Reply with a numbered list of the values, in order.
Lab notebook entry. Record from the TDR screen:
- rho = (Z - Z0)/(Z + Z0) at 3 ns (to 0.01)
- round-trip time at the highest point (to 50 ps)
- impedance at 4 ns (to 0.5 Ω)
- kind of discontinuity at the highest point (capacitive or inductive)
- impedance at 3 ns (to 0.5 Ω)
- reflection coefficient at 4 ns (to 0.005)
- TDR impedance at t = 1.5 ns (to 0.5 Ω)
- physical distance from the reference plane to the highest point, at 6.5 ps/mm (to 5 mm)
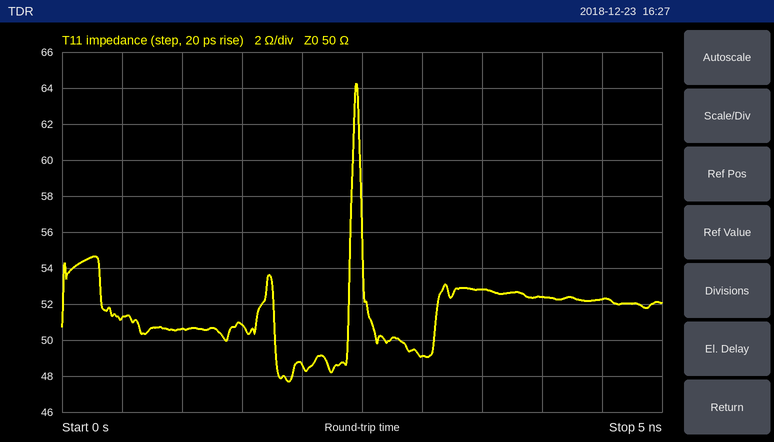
1. -0.01
2. 2.45 ns
3. 52.5 Ω
4. inductive
5. 49.0 Ω
6. +0.025
7. 51.0 Ω
8. 190 mm
